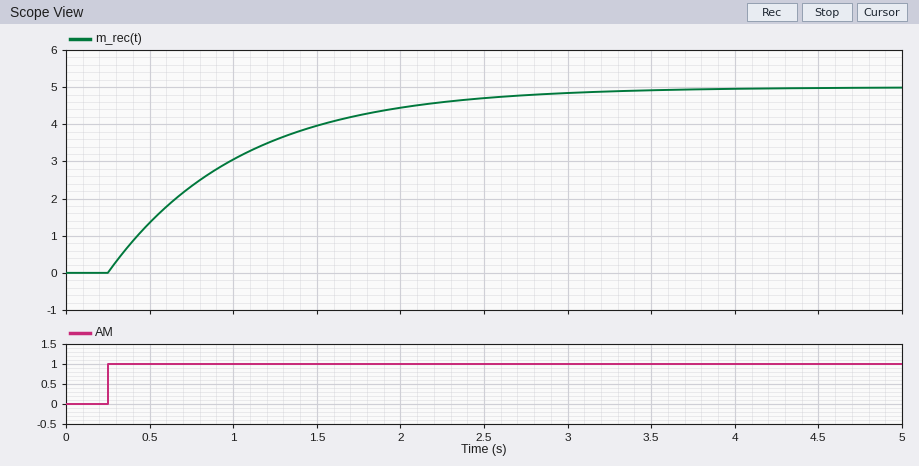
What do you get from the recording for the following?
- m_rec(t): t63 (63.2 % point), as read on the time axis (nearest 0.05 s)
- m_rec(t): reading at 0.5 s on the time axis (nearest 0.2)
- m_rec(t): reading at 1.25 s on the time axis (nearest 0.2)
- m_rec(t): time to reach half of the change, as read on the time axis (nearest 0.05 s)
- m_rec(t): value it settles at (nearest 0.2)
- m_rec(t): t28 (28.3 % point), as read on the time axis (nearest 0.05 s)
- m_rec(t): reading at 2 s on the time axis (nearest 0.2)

1.05 s
1.4
3.6
0.80 s
5.0
0.50 s
4.4
